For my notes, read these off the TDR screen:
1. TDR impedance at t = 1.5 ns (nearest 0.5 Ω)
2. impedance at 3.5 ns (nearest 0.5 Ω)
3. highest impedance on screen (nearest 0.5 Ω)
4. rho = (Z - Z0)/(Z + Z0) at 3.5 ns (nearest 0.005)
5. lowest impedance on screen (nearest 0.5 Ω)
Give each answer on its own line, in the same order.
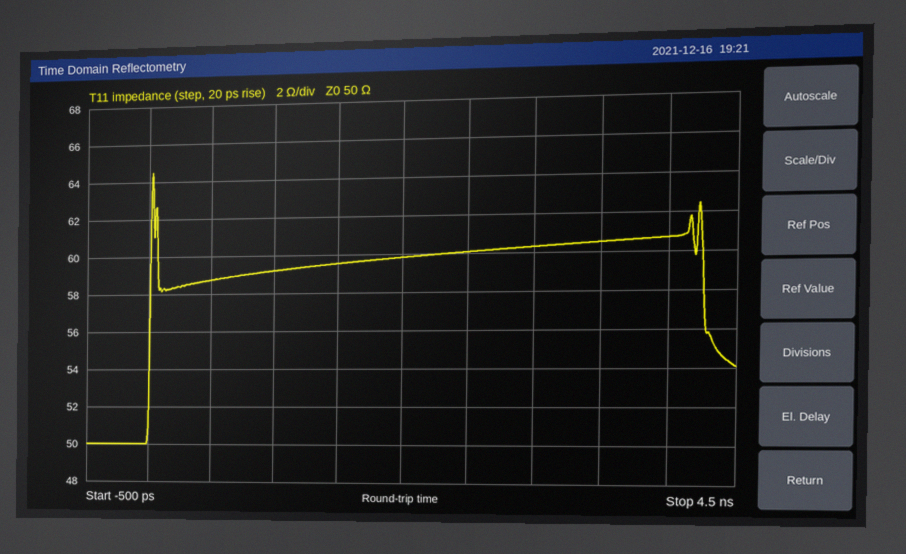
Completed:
59.5 Ω
60.5 Ω
64.5 Ω
+0.095
50.0 Ω
